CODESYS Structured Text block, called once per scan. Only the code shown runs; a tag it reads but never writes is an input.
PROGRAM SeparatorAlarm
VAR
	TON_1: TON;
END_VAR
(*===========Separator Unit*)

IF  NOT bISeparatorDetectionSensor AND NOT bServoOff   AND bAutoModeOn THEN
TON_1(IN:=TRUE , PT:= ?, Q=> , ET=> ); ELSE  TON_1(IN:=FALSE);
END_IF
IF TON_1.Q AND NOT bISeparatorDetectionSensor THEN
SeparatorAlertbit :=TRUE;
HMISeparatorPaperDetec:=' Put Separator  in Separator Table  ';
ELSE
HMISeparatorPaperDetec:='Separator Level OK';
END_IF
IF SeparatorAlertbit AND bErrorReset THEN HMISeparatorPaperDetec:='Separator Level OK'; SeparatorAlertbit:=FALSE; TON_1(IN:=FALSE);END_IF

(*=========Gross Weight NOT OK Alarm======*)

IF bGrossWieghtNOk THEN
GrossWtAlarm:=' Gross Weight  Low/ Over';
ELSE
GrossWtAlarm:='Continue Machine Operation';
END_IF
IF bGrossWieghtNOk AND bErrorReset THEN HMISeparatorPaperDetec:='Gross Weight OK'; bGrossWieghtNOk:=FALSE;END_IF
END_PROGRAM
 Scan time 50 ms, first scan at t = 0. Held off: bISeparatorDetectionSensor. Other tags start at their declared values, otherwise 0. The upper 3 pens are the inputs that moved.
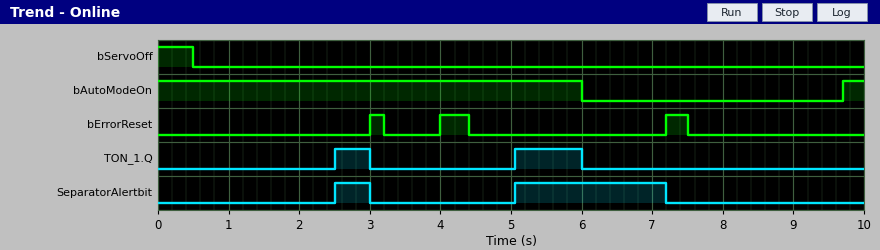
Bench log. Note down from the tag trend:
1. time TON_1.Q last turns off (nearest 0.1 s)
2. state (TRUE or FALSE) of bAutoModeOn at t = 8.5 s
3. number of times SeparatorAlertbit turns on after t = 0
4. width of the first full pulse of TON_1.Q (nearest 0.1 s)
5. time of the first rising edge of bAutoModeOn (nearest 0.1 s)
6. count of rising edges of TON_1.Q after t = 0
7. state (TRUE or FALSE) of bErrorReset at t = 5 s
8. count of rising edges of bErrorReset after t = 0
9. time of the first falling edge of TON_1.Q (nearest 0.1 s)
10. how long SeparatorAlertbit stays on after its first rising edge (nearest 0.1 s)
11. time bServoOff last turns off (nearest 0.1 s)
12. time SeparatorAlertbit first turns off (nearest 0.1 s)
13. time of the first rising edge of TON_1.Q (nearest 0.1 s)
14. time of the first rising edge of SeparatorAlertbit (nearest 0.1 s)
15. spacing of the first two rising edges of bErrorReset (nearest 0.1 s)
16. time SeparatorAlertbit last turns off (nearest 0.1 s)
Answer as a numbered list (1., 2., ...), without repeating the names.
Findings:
1. 6.0 s
2. FALSE
3. 2
4. 0.5 s
5. 9.7 s
6. 2
7. FALSE
8. 3
9. 3.0 s
10. 0.5 s
11. 0.5 s
12. 3.0 s
13. 2.5 s
14. 2.5 s
15. 1.0 s
16. 7.2 s
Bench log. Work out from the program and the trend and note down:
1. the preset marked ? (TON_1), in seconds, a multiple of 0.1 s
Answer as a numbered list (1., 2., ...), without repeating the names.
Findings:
1. 2.0 s
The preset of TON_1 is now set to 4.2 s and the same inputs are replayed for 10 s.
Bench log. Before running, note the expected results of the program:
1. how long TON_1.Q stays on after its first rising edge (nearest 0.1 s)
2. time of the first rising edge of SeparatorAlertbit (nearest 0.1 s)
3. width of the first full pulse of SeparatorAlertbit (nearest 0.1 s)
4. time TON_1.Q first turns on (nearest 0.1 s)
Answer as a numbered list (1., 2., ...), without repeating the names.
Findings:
1. 1.3 s
2. 4.7 s
3. 2.5 s
4. 4.7 s
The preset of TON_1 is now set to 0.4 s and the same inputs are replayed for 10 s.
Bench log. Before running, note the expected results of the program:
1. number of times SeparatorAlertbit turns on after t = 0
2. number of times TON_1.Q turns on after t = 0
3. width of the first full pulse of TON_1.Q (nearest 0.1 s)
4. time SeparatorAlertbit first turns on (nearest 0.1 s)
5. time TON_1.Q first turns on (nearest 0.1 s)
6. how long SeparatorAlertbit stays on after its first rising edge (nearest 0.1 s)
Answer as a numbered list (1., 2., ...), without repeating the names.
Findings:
1. 3
2. 3
3. 2.1 s
4. 0.9 s
5. 0.9 s
6. 2.1 s
